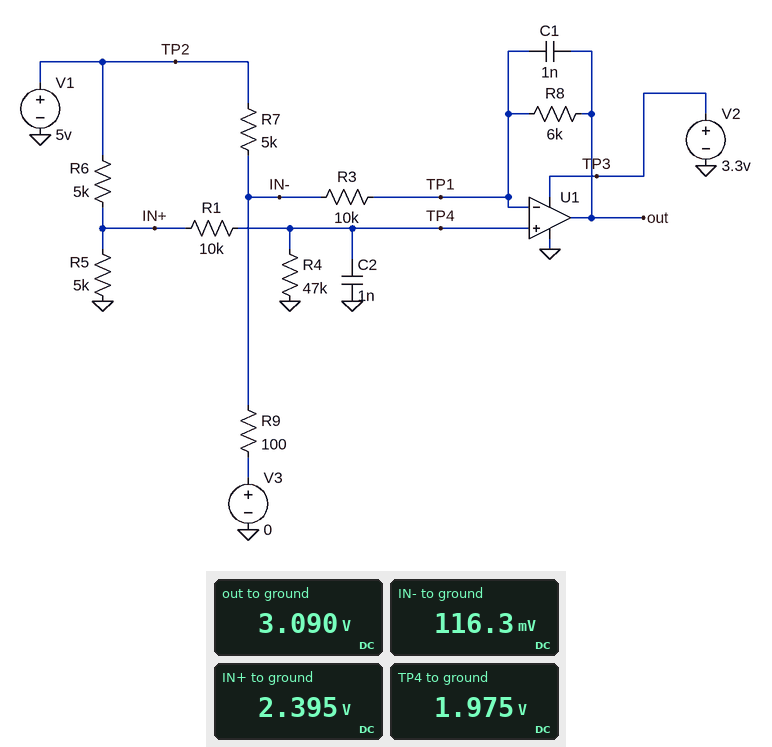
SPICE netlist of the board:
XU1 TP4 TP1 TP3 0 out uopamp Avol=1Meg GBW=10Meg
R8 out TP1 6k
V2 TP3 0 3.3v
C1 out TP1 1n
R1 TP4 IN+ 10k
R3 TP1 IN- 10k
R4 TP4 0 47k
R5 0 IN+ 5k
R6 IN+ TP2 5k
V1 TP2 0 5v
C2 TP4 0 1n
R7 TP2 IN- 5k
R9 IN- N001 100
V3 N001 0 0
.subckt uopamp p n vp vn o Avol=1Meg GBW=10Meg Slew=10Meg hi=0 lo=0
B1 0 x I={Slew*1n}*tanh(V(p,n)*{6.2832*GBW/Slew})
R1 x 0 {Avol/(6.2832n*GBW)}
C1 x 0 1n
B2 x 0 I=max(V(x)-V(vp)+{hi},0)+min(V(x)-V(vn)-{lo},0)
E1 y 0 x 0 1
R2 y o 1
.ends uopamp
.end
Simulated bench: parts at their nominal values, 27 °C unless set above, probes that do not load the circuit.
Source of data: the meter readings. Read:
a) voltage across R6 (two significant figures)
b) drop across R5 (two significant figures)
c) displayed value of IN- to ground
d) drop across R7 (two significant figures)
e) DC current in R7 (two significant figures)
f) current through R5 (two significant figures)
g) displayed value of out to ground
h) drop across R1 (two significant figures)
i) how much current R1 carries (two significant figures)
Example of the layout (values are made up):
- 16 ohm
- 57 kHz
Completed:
- 2.6 V
- 2.4 V
- 116.3 mV
- 4.9 V
- 980 µA
- 480 µA
- 3.090 V
- 420 mV
- 42 µA
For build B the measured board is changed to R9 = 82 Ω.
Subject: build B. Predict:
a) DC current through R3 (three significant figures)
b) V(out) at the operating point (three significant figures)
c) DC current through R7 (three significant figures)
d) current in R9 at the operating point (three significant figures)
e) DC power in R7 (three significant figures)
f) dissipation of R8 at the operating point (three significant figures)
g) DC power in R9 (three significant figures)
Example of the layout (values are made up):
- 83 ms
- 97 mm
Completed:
- 188 µA
- 3.10 V
- 981 µA
- 1.17 mA
- 4.81 mW
- 212 µW
- 112 µW
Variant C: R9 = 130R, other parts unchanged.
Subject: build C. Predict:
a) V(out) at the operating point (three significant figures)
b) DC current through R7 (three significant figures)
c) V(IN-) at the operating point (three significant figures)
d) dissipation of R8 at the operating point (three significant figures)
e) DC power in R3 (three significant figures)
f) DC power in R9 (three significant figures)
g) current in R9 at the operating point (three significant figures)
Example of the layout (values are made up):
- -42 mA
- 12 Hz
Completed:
- 3.07 V
- 970 µA
- 150 mV
- 200 µW
- 333 µW
- 173 µW
- 1.15 mA
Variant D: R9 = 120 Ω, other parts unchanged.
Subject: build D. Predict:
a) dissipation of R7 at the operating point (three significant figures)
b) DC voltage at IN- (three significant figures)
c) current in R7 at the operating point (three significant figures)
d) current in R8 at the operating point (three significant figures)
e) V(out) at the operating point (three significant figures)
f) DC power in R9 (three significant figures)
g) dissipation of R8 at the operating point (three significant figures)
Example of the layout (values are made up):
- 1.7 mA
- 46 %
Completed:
- 4.73 mW
- 139 mV
- 972 µA
- 184 µA
- 3.08 V
- 160 µW
- 202 µW
